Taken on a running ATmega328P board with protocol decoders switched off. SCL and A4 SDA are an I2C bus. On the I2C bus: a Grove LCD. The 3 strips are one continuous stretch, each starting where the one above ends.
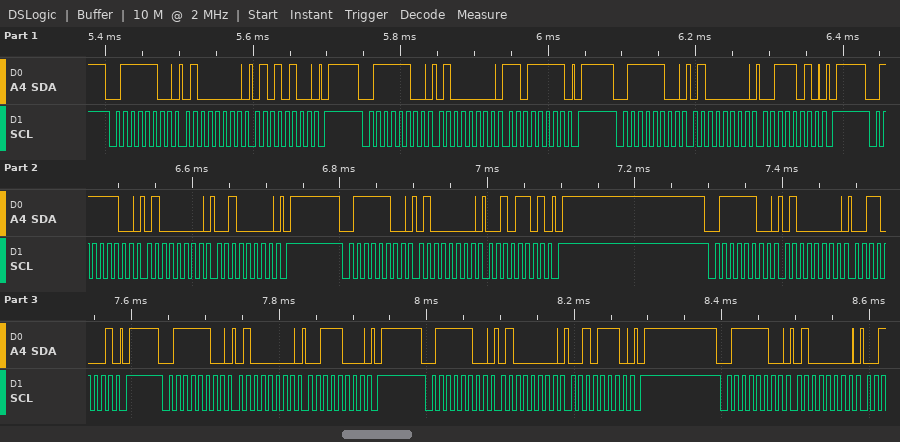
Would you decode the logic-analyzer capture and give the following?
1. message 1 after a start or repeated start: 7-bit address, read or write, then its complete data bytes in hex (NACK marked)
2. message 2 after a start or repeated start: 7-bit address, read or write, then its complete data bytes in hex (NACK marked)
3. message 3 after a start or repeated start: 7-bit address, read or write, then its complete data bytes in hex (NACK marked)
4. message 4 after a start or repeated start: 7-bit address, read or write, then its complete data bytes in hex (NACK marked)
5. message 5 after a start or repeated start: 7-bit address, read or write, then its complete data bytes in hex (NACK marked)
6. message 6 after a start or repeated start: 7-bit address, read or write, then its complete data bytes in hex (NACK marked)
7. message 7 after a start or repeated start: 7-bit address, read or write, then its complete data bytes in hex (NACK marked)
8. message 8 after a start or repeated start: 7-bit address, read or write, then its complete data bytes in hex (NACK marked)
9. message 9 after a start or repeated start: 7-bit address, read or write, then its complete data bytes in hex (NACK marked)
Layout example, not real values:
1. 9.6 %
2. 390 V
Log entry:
1. 0x3E write: 40 54
2. 0x3E write: 40 DF
3. 0x3E write: 40 3A
4. 0x3E write: 40 20
5. 0x3E write: 40 2D
6. 0x3E write: 40 31
7. 0x3E write: 40 38
8. 0x3E write: 40 2E
9. 0x3E write: 40
